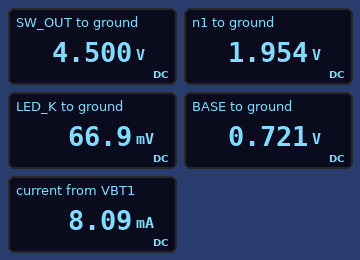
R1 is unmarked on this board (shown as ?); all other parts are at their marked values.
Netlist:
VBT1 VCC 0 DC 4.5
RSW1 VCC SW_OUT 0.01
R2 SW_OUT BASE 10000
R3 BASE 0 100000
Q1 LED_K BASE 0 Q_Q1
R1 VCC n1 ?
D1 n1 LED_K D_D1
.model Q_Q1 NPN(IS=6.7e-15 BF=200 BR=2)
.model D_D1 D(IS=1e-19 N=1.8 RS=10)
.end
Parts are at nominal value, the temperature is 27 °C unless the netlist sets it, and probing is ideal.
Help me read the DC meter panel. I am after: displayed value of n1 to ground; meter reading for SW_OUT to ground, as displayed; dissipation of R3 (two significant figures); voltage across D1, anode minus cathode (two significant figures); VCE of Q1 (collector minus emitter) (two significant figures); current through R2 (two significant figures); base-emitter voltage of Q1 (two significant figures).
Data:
1.954 V
4.500 V
5.2 µW
1.9 V
67 mV
380 µA
720 mV
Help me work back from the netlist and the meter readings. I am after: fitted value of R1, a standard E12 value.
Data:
330 Ω
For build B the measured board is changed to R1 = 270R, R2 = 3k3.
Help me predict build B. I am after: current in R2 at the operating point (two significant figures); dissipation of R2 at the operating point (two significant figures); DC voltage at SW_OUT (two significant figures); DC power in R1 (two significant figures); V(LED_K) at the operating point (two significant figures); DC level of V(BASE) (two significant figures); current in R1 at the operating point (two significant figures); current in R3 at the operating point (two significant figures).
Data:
1.1 mA
4.3 mW
4.5 V
24 mW
46 mV
730 mV
9.4 mA
7.3 µA
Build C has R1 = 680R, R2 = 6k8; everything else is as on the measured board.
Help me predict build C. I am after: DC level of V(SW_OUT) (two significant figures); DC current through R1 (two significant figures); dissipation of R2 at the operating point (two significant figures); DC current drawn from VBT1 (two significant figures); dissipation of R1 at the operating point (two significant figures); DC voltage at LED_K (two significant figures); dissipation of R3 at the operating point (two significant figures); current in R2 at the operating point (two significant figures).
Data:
4.5 V
3.9 mA
2.1 mW
4.4 mA
10 mW
43 mV
5.0 µW
560 µA
